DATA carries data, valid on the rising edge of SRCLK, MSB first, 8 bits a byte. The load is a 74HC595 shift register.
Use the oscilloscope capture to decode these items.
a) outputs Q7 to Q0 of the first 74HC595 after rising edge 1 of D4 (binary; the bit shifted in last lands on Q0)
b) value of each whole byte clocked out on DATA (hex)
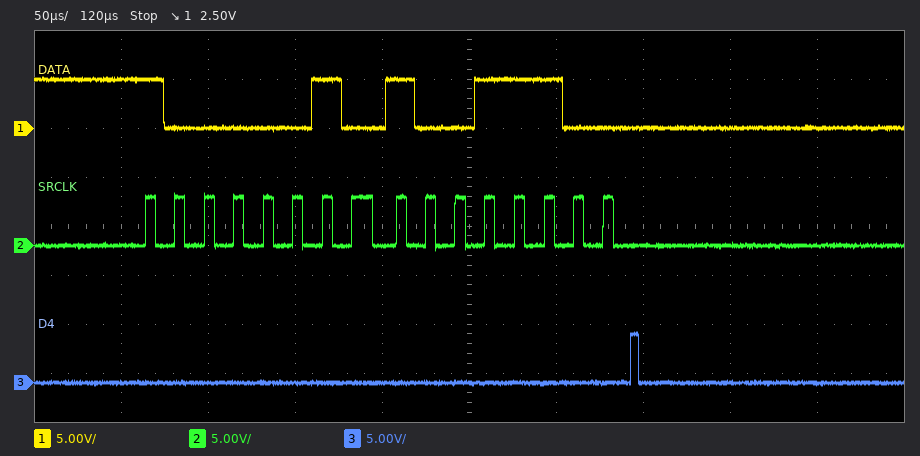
10011100
0x82 0x9C
